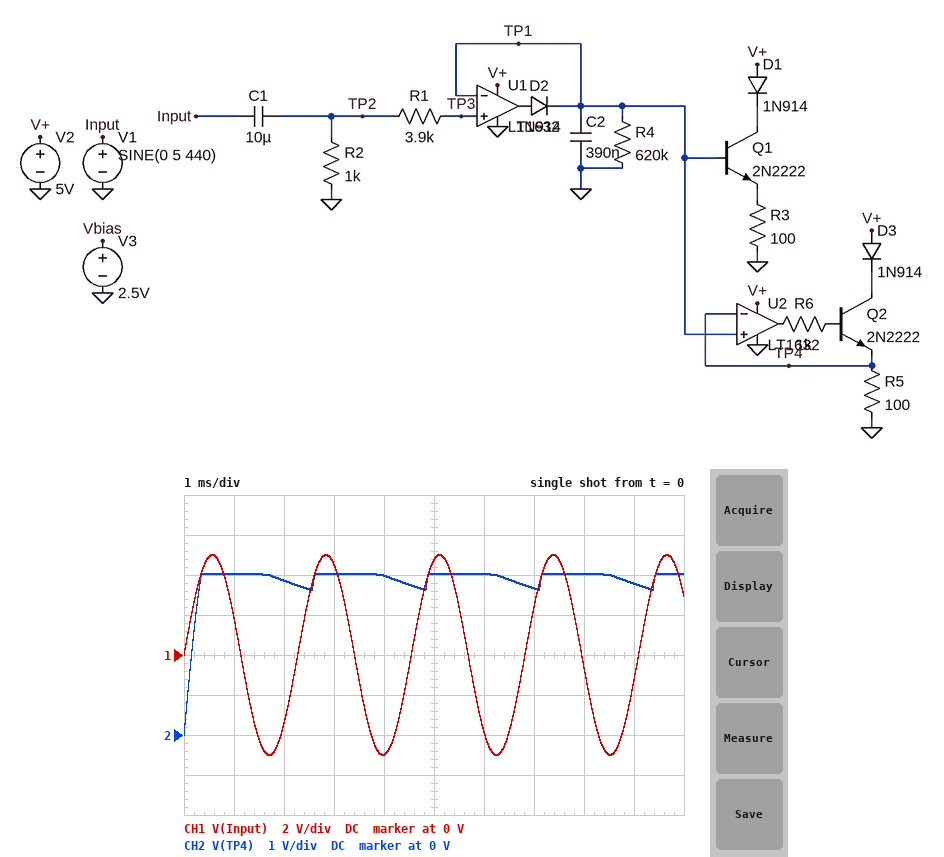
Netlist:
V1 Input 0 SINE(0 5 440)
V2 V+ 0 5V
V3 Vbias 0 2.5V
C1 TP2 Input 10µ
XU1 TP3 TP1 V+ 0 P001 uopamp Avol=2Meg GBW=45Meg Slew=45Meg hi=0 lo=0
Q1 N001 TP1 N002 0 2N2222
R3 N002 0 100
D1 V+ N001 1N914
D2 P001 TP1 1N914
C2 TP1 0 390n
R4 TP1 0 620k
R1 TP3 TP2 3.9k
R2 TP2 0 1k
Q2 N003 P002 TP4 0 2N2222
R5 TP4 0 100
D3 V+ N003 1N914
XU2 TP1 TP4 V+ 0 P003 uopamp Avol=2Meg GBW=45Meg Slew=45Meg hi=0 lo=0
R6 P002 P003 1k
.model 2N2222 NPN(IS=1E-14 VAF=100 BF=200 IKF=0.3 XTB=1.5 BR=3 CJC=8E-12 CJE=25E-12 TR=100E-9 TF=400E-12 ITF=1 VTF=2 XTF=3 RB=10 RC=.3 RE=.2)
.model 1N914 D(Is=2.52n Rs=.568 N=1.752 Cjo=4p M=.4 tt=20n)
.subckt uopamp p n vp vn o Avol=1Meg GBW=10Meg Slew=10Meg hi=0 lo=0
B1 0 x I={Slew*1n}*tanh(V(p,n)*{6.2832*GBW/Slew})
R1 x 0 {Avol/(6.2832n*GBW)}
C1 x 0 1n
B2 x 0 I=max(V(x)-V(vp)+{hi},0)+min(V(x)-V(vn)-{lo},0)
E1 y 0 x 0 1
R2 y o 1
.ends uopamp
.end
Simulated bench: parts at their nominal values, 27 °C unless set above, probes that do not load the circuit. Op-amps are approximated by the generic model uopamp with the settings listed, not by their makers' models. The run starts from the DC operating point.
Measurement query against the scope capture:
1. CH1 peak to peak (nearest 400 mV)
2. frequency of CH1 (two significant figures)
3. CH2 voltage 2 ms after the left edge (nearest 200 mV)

10.0 V
440 Hz
3.8 V
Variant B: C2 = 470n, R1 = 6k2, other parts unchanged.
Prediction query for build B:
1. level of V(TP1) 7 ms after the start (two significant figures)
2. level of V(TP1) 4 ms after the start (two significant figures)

3.8 V
4.1 V
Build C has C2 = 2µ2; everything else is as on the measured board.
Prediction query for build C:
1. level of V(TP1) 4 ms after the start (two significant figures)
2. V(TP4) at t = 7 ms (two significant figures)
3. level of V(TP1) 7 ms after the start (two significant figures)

4.4 V
4.0 V
4.3 V
